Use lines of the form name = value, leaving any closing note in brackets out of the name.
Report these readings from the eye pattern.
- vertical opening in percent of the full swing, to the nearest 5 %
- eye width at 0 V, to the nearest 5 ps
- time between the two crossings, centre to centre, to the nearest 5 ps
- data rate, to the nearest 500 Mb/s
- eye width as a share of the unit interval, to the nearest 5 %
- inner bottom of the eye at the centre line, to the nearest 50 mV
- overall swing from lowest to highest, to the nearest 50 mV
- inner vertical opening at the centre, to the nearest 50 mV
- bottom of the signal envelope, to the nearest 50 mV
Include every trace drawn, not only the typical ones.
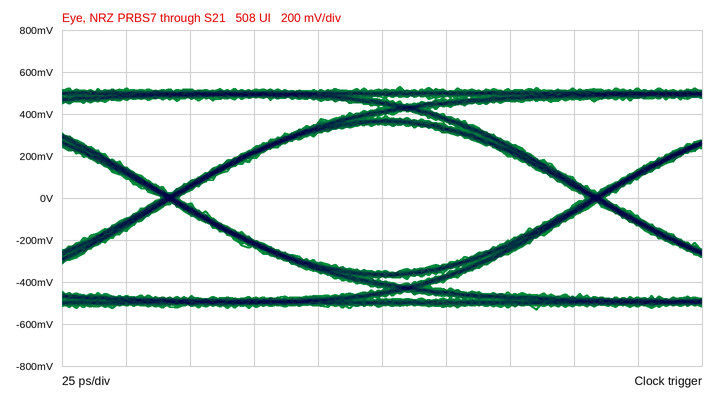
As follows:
vertical opening in percent of the full swing, to the nearest 5 % = 65 %
eye width at 0 V, to the nearest 5 ps = 160 ps
time between the two crossings, centre to centre, to the nearest 5 ps = 165 ps
data rate, to the nearest 500 Mb/s = 6.0 Gb/s
eye width as a share of the unit interval, to the nearest 5 % = 95 %
inner bottom of the eye at the centre line, to the nearest 50 mV = -350 mV
overall swing from lowest to highest, to the nearest 50 mV = 1.05 V
inner vertical opening at the centre, to the nearest 50 mV = 700 mV
bottom of the signal envelope, to the nearest 50 mV = -550 mV
